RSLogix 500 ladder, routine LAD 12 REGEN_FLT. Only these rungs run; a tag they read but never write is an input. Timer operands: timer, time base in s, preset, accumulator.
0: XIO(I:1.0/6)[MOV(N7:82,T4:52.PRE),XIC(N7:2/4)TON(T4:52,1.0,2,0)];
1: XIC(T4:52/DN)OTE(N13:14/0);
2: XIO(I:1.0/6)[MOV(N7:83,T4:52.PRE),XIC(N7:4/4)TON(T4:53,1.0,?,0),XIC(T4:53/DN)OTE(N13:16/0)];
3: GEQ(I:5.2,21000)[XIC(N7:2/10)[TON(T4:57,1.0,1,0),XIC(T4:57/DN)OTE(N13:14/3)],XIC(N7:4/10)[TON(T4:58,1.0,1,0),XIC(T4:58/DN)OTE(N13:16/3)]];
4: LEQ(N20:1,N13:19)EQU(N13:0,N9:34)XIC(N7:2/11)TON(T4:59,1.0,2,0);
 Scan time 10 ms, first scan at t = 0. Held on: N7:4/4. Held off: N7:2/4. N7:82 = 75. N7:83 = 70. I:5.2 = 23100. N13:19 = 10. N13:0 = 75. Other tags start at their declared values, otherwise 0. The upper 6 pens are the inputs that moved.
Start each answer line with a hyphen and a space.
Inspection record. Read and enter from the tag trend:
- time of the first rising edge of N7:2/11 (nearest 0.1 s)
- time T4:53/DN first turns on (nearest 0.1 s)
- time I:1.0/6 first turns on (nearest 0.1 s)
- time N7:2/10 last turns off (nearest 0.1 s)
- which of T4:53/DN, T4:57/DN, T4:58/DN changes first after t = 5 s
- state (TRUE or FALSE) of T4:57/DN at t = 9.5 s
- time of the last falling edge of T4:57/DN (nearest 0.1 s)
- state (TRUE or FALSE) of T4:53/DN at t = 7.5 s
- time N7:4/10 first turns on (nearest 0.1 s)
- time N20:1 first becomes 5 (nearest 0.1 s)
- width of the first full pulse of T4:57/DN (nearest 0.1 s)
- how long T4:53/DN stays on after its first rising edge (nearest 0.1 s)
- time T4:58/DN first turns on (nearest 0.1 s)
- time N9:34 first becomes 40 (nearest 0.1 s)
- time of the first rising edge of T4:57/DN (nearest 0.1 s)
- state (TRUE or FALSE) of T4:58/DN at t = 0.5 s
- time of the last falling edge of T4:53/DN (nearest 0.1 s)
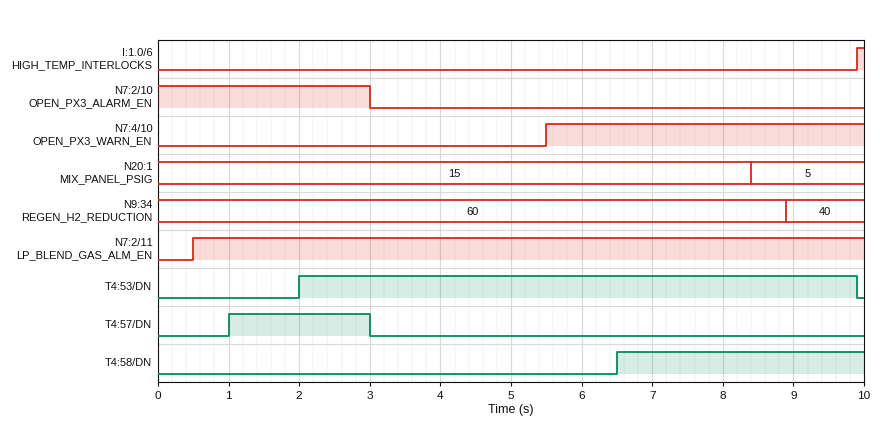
- 0.5 s
- 2.0 s
- 9.9 s
- 3.0 s
- T4:58/DN
- FALSE
- 3.0 s
- TRUE
- 5.5 s
- 8.4 s
- 2.0 s
- 7.9 s
- 6.5 s
- 8.9 s
- 1.0 s
- FALSE
- 9.9 s
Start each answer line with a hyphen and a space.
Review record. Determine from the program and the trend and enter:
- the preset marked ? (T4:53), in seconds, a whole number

- 2 s
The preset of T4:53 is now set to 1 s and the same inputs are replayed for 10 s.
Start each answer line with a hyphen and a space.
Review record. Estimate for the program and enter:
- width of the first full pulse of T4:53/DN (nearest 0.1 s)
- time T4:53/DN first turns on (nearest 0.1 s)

- 8.9 s
- 1.0 s
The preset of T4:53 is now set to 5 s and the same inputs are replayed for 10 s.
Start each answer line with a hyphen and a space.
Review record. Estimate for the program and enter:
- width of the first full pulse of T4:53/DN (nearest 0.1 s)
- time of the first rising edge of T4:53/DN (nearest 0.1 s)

- 4.9 s
- 5.0 s
